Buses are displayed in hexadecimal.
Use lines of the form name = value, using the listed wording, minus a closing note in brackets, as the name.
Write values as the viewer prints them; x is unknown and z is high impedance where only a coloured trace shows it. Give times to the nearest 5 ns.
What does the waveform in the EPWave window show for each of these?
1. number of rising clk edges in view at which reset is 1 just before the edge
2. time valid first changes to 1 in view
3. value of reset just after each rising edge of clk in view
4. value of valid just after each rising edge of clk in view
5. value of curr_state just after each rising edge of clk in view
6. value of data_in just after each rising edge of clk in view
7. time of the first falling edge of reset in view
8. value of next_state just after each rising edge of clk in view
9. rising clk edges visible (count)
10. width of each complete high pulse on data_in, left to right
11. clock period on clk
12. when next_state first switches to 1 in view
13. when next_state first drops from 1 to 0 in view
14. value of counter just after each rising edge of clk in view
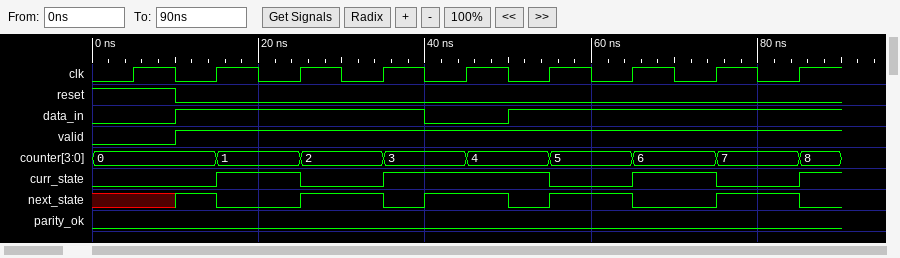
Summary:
number of rising clk edges in view at which reset is 1 just before the edge = 1
time valid first changes to 1 in view = 10 ns
value of reset just after each rising edge of clk in view = 1 0 0 0 0 0 0 0 0
value of valid just after each rising edge of clk in view = 0 1 1 1 1 1 1 1 1
value of curr_state just after each rising edge of clk in view = 0 1 0 1 1 0 1 0 1
value of data_in just after each rising edge of clk in view = 0 1 1 1 0 1 1 1 1
time of the first falling edge of reset in view = 10 ns
value of next_state just after each rising edge of clk in view = x 0 1 0 1 1 0 1 0
rising clk edges visible = 9
width of each complete high pulse on data_in, left to right = 30 ns
clock period on clk = 10 ns
when next_state first switches to 1 in view = 10 ns
when next_state first drops from 1 to 0 in view = 15 ns
value of counter just after each rising edge of clk in view = 0, 1, 2, 3, 4, 5, 6, 7, 8
